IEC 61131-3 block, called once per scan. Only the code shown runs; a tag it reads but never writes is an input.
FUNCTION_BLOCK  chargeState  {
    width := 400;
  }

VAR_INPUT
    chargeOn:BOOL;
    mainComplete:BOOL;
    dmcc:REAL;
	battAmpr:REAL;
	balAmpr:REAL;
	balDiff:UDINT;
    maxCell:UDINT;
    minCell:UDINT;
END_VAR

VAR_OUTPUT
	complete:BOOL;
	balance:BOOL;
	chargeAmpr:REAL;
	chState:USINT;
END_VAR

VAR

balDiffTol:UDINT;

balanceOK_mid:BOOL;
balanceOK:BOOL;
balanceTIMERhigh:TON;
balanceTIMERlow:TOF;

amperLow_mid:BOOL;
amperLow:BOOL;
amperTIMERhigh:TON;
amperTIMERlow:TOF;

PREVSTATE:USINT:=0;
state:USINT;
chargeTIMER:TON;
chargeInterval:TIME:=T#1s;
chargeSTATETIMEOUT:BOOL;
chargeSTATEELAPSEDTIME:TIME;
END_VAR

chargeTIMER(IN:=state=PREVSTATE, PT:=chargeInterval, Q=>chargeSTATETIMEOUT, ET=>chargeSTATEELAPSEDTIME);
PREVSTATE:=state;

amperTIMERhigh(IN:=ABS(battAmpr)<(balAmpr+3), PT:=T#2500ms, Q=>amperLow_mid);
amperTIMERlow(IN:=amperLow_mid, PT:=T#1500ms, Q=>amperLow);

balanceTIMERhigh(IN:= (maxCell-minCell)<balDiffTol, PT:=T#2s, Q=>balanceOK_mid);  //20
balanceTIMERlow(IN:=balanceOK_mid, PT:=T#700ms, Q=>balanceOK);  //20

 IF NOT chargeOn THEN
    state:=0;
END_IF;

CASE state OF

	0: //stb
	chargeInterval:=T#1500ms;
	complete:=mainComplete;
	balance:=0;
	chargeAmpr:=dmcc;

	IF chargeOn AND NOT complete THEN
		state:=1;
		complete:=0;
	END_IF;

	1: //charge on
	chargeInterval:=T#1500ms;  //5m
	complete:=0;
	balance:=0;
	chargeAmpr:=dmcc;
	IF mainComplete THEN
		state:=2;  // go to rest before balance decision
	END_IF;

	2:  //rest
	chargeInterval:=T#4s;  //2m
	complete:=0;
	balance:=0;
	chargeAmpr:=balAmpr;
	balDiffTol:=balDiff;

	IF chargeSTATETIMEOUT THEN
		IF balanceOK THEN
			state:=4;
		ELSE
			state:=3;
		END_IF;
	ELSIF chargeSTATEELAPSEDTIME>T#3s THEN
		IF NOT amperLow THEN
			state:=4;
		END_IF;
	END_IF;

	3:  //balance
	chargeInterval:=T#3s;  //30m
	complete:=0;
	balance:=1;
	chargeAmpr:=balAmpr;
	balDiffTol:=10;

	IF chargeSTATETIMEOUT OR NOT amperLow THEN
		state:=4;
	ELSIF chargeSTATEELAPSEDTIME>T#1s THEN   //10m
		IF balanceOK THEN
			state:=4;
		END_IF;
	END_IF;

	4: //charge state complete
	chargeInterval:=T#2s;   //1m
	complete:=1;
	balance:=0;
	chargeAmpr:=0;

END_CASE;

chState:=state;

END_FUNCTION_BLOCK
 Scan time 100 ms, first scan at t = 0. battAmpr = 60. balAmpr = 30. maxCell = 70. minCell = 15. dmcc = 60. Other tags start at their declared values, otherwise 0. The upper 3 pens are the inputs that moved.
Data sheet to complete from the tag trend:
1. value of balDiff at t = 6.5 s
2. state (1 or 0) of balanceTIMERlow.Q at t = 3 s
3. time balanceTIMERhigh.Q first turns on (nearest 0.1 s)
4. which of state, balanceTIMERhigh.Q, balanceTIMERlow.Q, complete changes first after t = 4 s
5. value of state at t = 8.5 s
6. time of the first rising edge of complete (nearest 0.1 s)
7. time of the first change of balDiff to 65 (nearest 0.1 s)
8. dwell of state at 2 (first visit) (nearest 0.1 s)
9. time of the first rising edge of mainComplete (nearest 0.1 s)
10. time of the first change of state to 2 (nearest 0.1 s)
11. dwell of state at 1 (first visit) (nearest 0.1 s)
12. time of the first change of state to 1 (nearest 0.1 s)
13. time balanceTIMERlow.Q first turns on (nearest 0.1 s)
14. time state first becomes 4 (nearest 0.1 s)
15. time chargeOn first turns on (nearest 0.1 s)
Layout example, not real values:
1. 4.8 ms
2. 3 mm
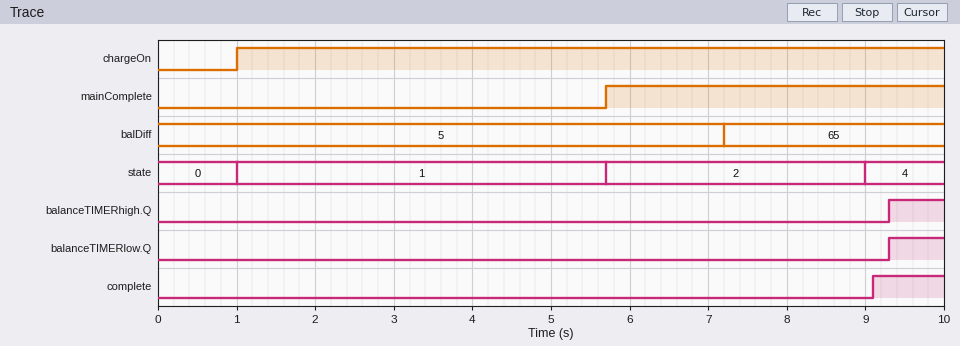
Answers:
1. 5
2. 0
3. 9.3 s
4. state
5. 2
6. 9.1 s
7. 7.2 s
8. 3.3 s
9. 5.7 s
10. 5.7 s
11. 4.7 s
12. 1.0 s
13. 9.3 s
14. 9.0 s
15. 1.0 s
